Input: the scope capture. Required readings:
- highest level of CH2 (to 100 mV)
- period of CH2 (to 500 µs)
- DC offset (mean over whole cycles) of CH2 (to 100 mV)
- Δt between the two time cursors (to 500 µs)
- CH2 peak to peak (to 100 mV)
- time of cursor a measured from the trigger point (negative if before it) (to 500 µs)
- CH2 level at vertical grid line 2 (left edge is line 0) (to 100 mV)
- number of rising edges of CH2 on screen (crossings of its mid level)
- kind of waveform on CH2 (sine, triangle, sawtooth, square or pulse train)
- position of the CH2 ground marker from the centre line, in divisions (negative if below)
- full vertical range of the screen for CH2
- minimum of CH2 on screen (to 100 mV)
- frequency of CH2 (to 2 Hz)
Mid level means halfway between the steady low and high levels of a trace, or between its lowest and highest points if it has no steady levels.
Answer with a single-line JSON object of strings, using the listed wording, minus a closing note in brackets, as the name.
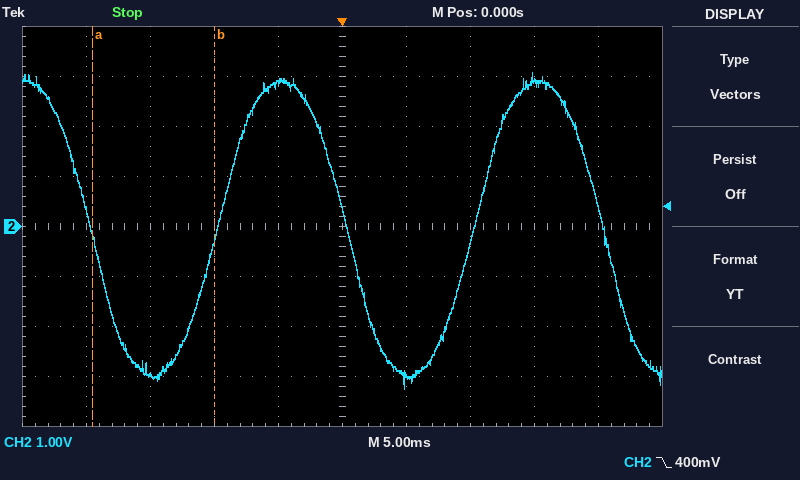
{"highest level of CH2": "3.1 V", "period of CH2": "20.0 ms", "DC offset (mean over whole cycles) of CH2": "0.0 V", "Δt between the two time cursors": "9.5 ms", "CH2 peak to peak": "6.3 V", "time of cursor a measured from the trigger point (negative if before it)": "-19.5 ms", "CH2 level at vertical grid line 2 (left edge is line 0)": "-3.0 V", "number of rising edges of CH2 on screen": "2", "kind of waveform on CH2": "sine", "position of the CH2 ground marker from the centre line, in divisions": "0.0 div", "full vertical range of the screen for CH2": "8 V", "minimum of CH2 on screen": "-3.2 V", "frequency of CH2": "50 Hz"}
